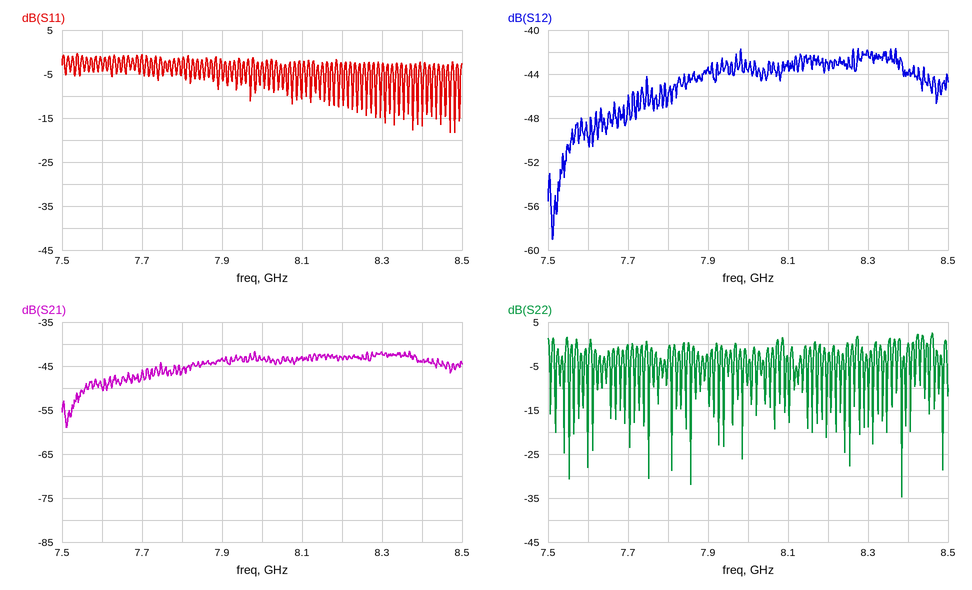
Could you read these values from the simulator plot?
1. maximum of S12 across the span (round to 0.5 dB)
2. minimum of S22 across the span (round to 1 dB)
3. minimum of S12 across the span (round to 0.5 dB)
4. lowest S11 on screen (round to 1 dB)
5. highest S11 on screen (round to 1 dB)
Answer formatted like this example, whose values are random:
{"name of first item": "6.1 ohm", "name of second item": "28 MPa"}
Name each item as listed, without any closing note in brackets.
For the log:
{"maximum of S12 across the span": "-41.5 dB", "minimum of S22 across the span": "-35 dB", "minimum of S12 across the span": "-59.0 dB", "lowest S11 on screen": "-18 dB", "highest S11 on screen": "0 dB"}
